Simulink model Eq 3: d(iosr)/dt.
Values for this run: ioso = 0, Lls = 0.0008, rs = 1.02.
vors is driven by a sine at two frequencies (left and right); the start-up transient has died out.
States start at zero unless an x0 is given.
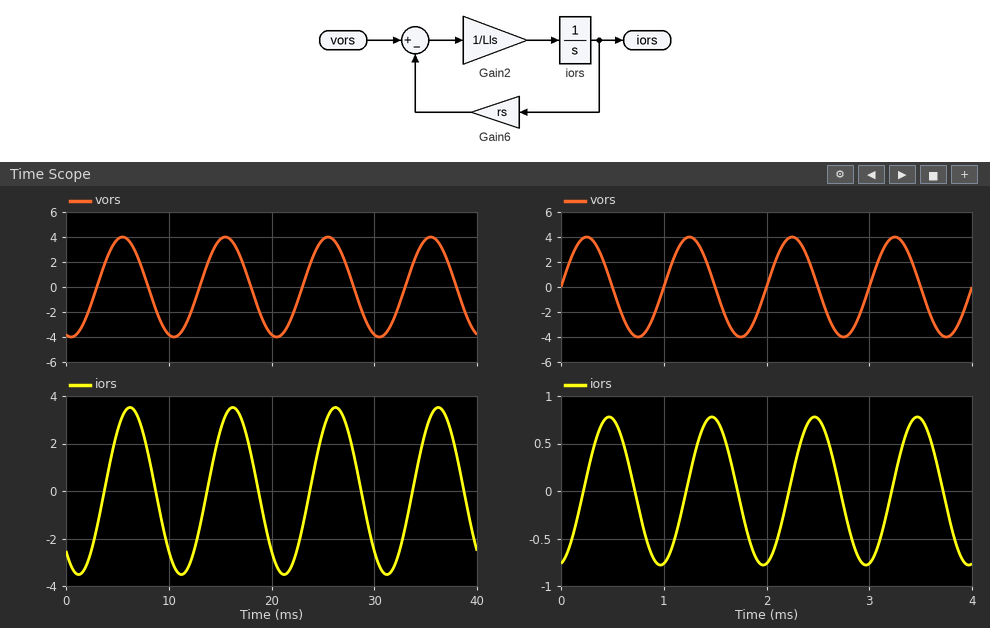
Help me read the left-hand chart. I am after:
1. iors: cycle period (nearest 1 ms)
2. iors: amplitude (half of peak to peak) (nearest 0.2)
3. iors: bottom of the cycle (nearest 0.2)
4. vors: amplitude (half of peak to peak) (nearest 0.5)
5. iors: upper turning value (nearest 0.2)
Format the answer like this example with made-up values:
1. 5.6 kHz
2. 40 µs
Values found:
1. 10 ms
2. 3.6
3. -3.6
4. 4.0
5. 3.6
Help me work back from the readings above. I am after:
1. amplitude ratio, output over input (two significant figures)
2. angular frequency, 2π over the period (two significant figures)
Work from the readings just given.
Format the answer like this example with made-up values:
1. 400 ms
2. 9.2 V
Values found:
1. 0.90
2. 0.63 rad/ms
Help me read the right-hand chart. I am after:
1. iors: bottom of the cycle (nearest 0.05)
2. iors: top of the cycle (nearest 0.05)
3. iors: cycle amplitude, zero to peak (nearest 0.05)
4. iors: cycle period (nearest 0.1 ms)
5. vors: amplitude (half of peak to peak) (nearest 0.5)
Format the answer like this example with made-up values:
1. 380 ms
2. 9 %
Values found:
1. -0.80
2. 0.80
3. 0.80
4. 1.0 ms
5. 4.0
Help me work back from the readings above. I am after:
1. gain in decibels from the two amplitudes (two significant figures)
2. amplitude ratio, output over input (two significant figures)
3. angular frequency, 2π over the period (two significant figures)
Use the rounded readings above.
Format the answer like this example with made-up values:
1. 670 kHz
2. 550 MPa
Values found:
1. -14 dB
2. 0.20
3. 6.3 rad/ms
